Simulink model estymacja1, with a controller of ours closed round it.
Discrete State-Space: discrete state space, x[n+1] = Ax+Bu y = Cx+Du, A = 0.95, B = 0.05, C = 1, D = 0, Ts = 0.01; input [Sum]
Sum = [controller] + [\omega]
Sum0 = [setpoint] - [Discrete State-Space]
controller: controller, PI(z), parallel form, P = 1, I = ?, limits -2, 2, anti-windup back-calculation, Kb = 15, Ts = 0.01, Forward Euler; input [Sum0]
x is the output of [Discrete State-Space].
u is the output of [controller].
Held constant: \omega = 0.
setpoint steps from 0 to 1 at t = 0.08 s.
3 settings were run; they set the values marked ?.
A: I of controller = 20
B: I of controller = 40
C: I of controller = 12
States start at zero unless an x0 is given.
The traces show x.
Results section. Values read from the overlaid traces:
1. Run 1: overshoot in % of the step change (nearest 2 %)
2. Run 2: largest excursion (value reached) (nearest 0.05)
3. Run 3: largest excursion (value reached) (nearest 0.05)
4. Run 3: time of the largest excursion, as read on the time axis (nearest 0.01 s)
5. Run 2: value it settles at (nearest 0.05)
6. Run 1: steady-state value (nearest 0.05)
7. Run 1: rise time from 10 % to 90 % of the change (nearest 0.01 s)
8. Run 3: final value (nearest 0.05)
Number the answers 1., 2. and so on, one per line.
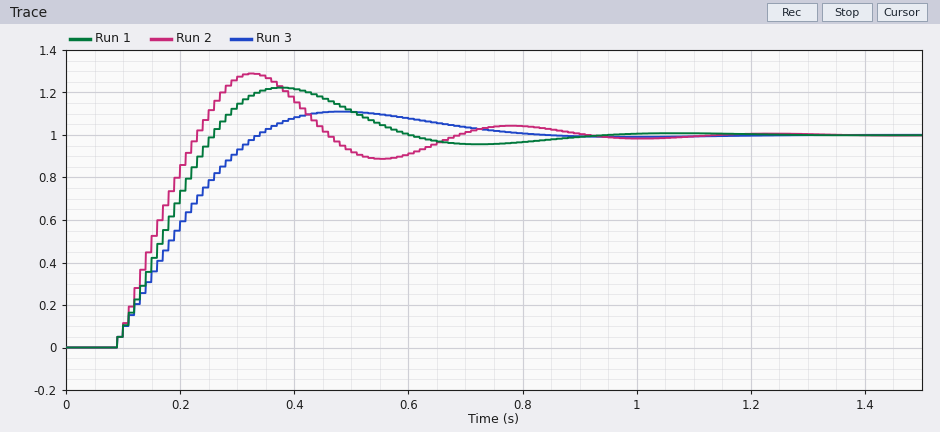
1. 22 %
2. 1.30
3. 1.10
4. 0.48 s
5. 1.00
6. 1.00
7. 0.14 s
8. 1.00
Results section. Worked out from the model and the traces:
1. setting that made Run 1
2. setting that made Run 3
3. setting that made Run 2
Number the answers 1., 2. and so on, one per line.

1. A
2. C
3. B
